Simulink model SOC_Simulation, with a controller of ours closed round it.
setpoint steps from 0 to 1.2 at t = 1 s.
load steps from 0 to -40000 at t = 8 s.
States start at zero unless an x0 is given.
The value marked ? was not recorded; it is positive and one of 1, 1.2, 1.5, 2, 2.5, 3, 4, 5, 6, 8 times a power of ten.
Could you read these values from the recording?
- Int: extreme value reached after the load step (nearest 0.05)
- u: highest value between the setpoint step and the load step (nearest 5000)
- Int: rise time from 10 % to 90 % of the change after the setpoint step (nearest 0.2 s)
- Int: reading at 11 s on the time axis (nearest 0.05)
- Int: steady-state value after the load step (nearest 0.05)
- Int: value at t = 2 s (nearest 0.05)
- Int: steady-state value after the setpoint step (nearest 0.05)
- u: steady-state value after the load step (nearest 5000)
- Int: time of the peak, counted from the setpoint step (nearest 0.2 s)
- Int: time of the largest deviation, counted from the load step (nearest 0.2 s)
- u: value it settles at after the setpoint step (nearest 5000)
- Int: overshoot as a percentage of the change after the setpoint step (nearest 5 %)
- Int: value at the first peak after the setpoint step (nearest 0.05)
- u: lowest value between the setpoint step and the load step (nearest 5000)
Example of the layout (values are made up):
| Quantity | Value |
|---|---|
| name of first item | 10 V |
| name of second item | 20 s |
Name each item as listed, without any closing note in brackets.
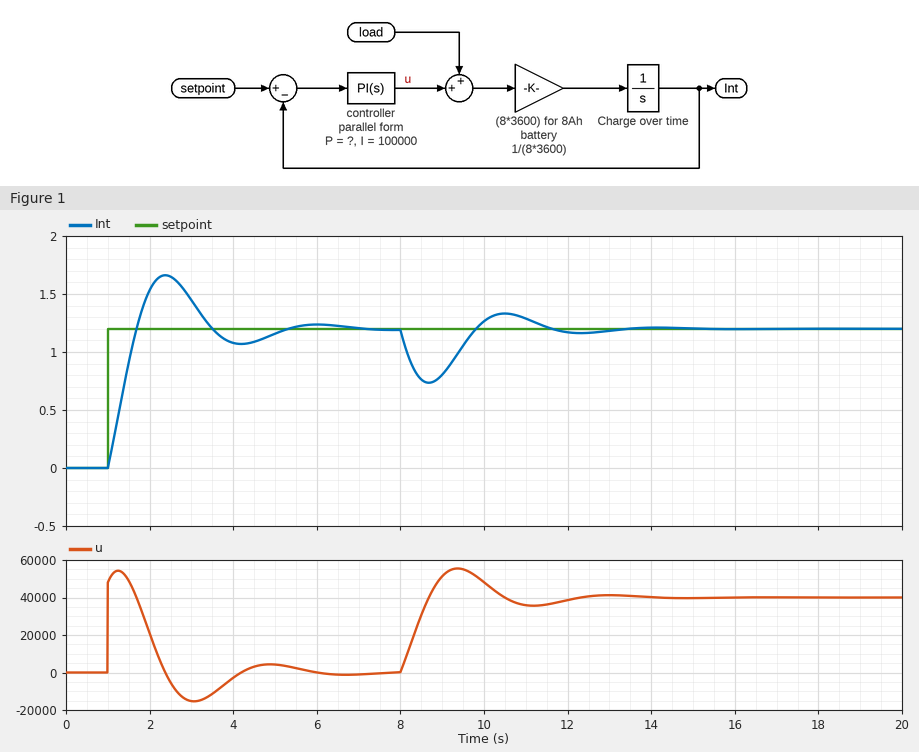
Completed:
| Quantity | Value |
|---|---|
| Int: extreme value reached after the load step | 0.75 |
| u: highest value between the setpoint step and the load step | 55000 |
| Int: rise time from 10 % to 90 % of the change after the setpoint step | 0.6 s |
| Int: reading at 11 s on the time axis | 1.30 |
| Int: steady-state value after the load step | 1.20 |
| Int: value at t = 2 s | 1.55 |
| Int: steady-state value after the setpoint step | 1.20 |
| u: steady-state value after the load step | 40000 |
| Int: time of the peak, counted from the setpoint step | 1.4 s |
| Int: time of the largest deviation, counted from the load step | 0.6 s |
| u: value it settles at after the setpoint step | 0 |
| Int: overshoot as a percentage of the change after the setpoint step | 40 % |
| Int: value at the first peak after the setpoint step | 1.65 |
| u: lowest value between the setpoint step and the load step | -15000 |
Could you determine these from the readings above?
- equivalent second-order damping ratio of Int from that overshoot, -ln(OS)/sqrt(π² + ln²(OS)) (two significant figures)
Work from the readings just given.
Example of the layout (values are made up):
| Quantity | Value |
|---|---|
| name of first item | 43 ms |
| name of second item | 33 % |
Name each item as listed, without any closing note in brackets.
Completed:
| Quantity | Value |
|---|---|
| equivalent second-order damping ratio of Int from that overshoot, -ln(OS)/sqrt(π² + ln²(OS)) | 0.28 |
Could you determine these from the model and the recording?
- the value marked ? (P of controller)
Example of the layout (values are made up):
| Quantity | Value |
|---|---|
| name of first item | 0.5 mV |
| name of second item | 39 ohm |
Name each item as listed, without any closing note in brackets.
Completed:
| Quantity | Value |
|---|---|
| the value marked ? | 40000 |
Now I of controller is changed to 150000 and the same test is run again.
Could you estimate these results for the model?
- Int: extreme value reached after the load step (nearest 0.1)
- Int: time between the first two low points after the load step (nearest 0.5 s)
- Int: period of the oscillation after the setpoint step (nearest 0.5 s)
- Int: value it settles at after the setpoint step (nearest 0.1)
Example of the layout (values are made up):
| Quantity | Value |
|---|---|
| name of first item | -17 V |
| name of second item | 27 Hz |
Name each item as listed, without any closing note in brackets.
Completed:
| Quantity | Value |
|---|---|
| Int: extreme value reached after the load step | 0.8 |
| Int: time between the first two low points after the load step | 3.0 s |
| Int: period of the oscillation after the setpoint step | 3.0 s |
| Int: value it settles at after the setpoint step | 1.2 |
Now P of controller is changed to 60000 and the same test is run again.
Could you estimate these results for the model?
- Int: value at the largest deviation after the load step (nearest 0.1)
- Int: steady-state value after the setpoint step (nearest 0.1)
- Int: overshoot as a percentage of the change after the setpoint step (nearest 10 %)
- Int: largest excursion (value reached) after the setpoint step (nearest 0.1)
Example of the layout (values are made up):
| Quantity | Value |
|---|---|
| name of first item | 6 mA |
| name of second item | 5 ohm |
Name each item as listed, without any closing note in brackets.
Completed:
| Quantity | Value |
|---|---|
| Int: value at the largest deviation after the load step | 0.8 |
| Int: steady-state value after the setpoint step | 1.2 |
| Int: overshoot as a percentage of the change after the setpoint step | 30 % |
| Int: largest excursion (value reached) after the setpoint step | 1.5 |
